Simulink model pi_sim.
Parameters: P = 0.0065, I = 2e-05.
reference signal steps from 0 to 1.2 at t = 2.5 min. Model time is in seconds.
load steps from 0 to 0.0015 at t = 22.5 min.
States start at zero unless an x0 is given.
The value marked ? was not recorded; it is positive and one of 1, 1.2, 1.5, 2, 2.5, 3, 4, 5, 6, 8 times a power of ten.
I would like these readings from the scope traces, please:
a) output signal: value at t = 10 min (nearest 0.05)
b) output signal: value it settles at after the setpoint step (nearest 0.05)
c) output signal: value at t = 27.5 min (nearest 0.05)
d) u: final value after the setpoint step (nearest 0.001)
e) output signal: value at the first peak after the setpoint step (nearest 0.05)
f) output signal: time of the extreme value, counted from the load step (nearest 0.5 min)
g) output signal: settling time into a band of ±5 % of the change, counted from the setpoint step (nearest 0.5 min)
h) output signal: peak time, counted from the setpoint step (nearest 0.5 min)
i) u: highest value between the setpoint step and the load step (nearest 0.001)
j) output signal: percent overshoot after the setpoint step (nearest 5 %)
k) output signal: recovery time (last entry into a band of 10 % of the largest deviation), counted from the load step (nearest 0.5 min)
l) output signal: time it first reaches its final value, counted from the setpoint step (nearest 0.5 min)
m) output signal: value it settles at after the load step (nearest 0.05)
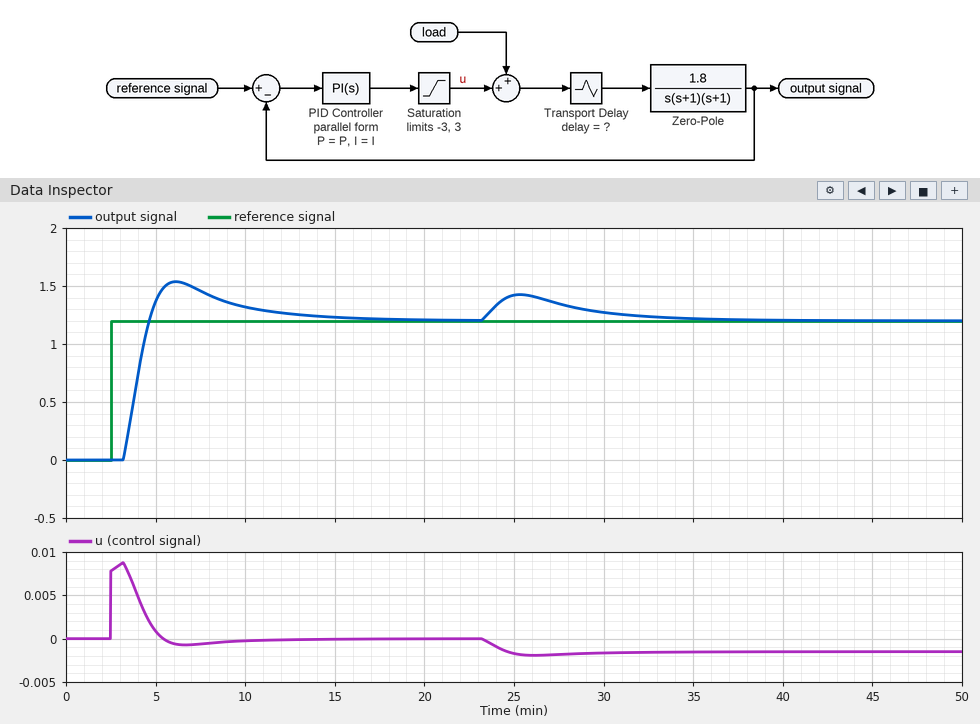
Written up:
1.30
1.20
1.35
0.000
1.55
3.0 min
10.0 min
3.5 min
0.009
30 %
12.0 min
2.0 min
1.20
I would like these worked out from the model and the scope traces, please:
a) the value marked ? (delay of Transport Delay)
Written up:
40
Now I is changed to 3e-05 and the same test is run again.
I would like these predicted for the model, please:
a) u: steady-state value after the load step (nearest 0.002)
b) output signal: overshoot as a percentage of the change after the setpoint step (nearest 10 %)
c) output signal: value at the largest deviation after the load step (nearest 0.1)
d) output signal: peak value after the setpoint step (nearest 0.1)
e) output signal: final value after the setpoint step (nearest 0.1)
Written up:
-0.002
40 %
1.4
1.7
1.2
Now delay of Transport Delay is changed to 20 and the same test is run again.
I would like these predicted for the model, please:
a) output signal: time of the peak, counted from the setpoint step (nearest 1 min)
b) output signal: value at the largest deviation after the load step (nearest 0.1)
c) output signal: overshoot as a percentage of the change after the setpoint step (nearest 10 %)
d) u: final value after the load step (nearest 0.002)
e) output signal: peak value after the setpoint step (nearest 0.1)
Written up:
5 min
1.4
20 %
-0.002
1.4
